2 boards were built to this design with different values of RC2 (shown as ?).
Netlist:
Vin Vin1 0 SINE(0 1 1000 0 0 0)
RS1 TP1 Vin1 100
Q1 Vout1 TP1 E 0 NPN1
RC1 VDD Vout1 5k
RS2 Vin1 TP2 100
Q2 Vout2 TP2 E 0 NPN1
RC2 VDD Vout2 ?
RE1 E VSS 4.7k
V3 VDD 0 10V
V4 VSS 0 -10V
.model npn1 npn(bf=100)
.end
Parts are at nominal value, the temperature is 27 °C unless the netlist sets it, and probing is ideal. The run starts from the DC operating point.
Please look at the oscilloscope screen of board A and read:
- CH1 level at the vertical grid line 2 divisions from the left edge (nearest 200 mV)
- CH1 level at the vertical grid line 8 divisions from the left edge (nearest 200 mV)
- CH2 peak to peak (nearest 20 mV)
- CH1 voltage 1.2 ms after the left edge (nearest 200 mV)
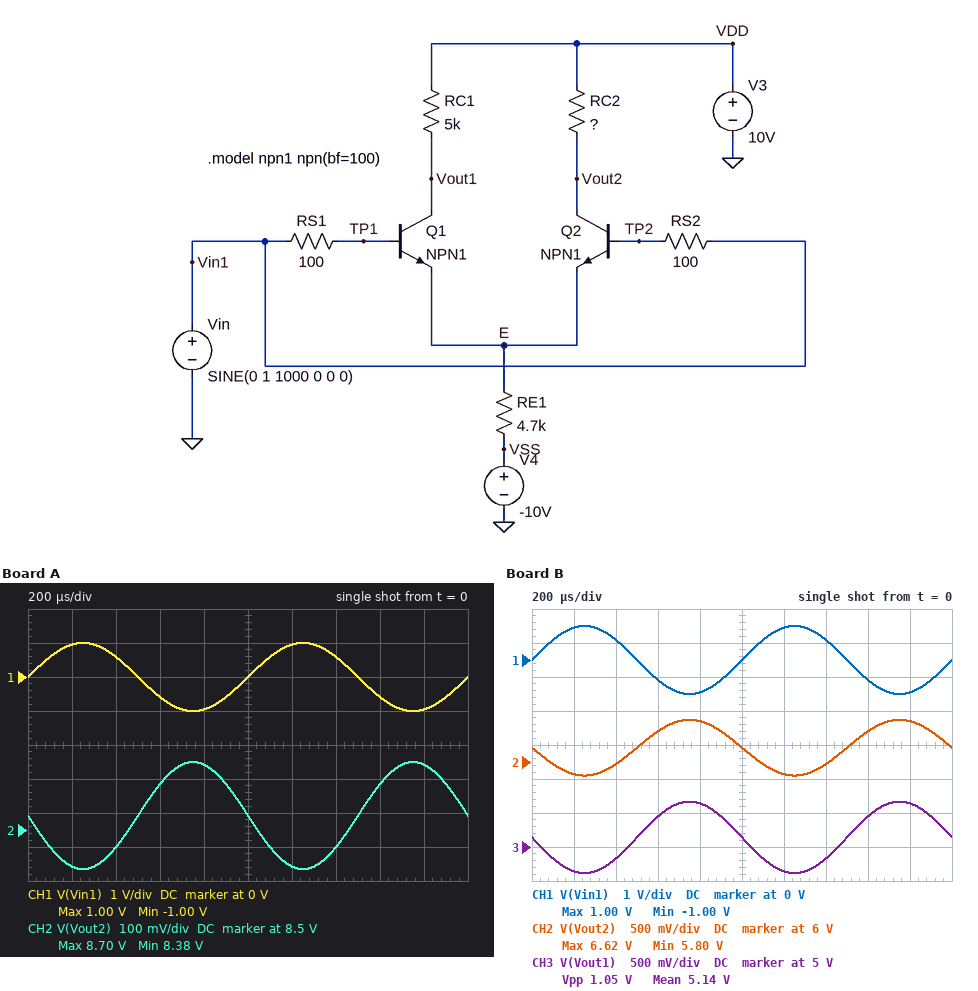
600 mV
-600 mV
320 mV
1.0 V
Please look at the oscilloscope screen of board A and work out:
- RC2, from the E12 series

1.5 kΩ
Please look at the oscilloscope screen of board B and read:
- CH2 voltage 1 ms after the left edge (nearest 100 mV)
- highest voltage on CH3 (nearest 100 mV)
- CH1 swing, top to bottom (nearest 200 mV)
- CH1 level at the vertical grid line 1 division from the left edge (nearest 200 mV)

6.2 V
5.7 V
2.0 V
1.0 V
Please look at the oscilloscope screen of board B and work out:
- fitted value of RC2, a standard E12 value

3.9 kΩ
